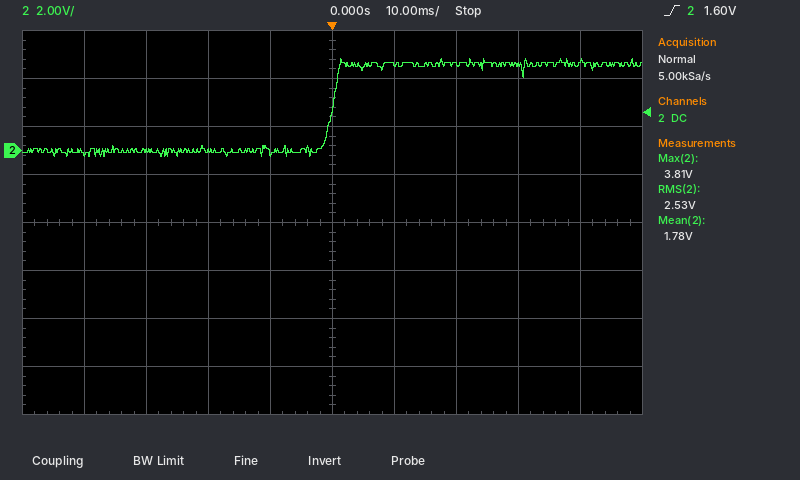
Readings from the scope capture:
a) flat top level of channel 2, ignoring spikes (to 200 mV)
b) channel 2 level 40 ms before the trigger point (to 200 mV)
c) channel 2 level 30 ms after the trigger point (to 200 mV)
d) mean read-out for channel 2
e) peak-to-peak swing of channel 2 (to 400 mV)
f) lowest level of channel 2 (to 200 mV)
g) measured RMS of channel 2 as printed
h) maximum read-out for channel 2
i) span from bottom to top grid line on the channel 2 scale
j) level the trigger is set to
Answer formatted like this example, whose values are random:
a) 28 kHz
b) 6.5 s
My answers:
a) 3.6 V
b) -200 mV
c) 3.6 V
d) 1.78 V
e) 4.0 V
f) -200 mV
g) 2.53 V
h) 3.81 V
i) 16 V
j) 1.60 V
